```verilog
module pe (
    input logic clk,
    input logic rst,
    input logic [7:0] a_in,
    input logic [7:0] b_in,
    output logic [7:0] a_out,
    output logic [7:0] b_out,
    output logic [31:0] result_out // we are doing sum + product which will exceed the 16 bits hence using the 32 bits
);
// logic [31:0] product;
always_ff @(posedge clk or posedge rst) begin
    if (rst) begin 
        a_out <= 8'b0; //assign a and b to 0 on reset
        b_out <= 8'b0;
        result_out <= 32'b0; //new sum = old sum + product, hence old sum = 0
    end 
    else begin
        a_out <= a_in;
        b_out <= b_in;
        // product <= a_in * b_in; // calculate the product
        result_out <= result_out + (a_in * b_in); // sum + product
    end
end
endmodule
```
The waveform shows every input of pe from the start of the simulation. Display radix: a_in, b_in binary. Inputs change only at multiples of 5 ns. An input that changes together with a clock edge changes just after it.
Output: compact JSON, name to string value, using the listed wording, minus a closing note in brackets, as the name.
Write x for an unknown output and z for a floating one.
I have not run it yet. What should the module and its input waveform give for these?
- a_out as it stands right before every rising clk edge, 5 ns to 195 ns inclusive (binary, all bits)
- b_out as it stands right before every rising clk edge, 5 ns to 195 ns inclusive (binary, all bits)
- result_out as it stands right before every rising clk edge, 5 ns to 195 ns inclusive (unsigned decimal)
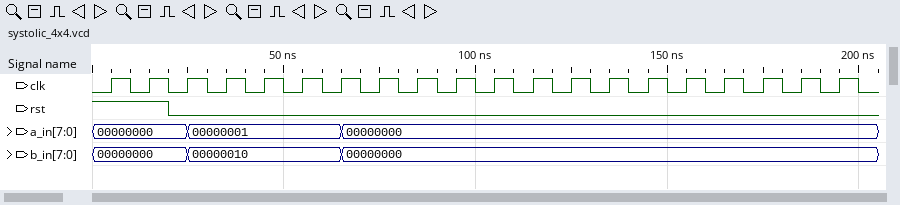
{"a_out as it stands right before every rising clk edge, 5 ns to 195 ns inclusive": "00000000, 00000000, 00000000, 00000000, 00000001, 00000001, 00000001, 00000001, 00000000, 00000000, 00000000, 00000000, 00000000, 00000000, 00000000, 00000000, 00000000, 00000000, 00000000, 00000000", "b_out as it stands right before every rising clk edge, 5 ns to 195 ns inclusive": "00000000, 00000000, 00000000, 00000000, 00000010, 00000010, 00000010, 00000010, 00000000, 00000000, 00000000, 00000000, 00000000, 00000000, 00000000, 00000000, 00000000, 00000000, 00000000, 00000000", "result_out as it stands right before every rising clk edge, 5 ns to 195 ns inclusive": "0, 0, 0, 0, 2, 4, 6, 8, 8, 8, 8, 8, 8, 8, 8, 8, 8, 8, 8, 8"}
